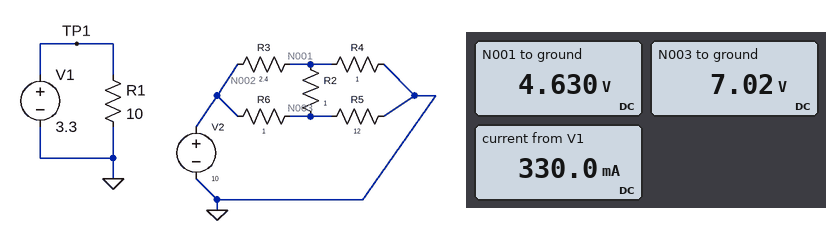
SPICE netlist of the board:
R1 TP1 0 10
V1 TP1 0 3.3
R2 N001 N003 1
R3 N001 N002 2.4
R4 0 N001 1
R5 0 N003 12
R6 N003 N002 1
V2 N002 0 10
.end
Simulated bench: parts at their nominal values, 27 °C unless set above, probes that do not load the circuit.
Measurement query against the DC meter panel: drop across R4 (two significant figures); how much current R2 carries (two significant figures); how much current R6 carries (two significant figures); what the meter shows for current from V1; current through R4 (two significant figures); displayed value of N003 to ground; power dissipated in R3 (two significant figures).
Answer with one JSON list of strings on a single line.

["4.6 V", "2.4 A", "3.0 A", "330.0 mA", "4.6 A", "7.02 V", "12 W"]
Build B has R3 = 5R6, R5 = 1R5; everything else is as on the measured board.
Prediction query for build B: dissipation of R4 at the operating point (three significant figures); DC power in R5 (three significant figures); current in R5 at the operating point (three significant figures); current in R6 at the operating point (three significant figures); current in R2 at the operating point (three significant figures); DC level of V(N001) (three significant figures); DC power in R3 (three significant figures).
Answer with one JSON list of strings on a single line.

["9.42 W", "16.0 W", "3.27 A", "5.10 A", "1.83 A", "3.07 V", "8.58 W"]
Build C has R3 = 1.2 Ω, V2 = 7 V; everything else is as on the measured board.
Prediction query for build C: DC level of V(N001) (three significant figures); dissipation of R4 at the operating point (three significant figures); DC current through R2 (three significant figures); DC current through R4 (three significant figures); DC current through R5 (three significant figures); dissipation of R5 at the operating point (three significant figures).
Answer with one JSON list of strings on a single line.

["3.91 V", "15.3 W", "1.33 A", "3.91 A", "436 mA", "2.28 W"]
